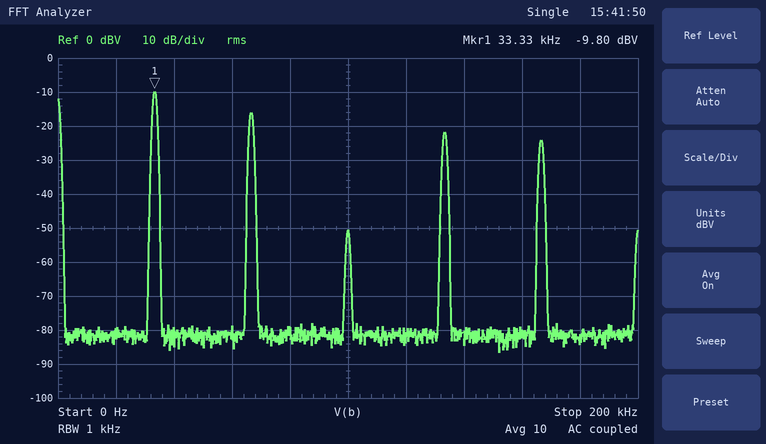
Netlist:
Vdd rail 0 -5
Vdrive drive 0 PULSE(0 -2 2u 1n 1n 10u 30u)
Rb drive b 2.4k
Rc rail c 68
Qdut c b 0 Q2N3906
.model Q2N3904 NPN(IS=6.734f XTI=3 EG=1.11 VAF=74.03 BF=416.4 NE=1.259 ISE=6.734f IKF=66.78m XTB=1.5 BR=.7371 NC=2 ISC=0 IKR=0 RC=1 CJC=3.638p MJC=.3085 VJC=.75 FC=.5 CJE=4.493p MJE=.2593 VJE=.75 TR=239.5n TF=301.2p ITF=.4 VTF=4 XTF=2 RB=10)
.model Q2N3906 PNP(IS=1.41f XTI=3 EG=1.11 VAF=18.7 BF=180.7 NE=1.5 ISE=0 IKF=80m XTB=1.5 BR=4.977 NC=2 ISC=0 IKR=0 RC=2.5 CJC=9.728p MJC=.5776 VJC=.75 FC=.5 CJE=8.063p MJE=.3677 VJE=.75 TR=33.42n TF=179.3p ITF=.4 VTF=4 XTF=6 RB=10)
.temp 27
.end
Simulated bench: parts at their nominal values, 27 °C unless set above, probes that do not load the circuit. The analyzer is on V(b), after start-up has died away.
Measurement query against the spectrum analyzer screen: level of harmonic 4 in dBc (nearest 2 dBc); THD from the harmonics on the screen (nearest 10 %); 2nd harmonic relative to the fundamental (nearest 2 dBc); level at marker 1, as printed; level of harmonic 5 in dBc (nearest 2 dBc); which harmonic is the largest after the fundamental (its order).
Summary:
-12 dBc
60 %
-6 dBc
-9.80 dBV
-14 dBc
2
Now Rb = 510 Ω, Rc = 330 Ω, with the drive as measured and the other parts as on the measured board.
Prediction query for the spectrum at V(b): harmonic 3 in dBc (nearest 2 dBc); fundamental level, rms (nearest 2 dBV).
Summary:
-34 dBc
-10 dBV
